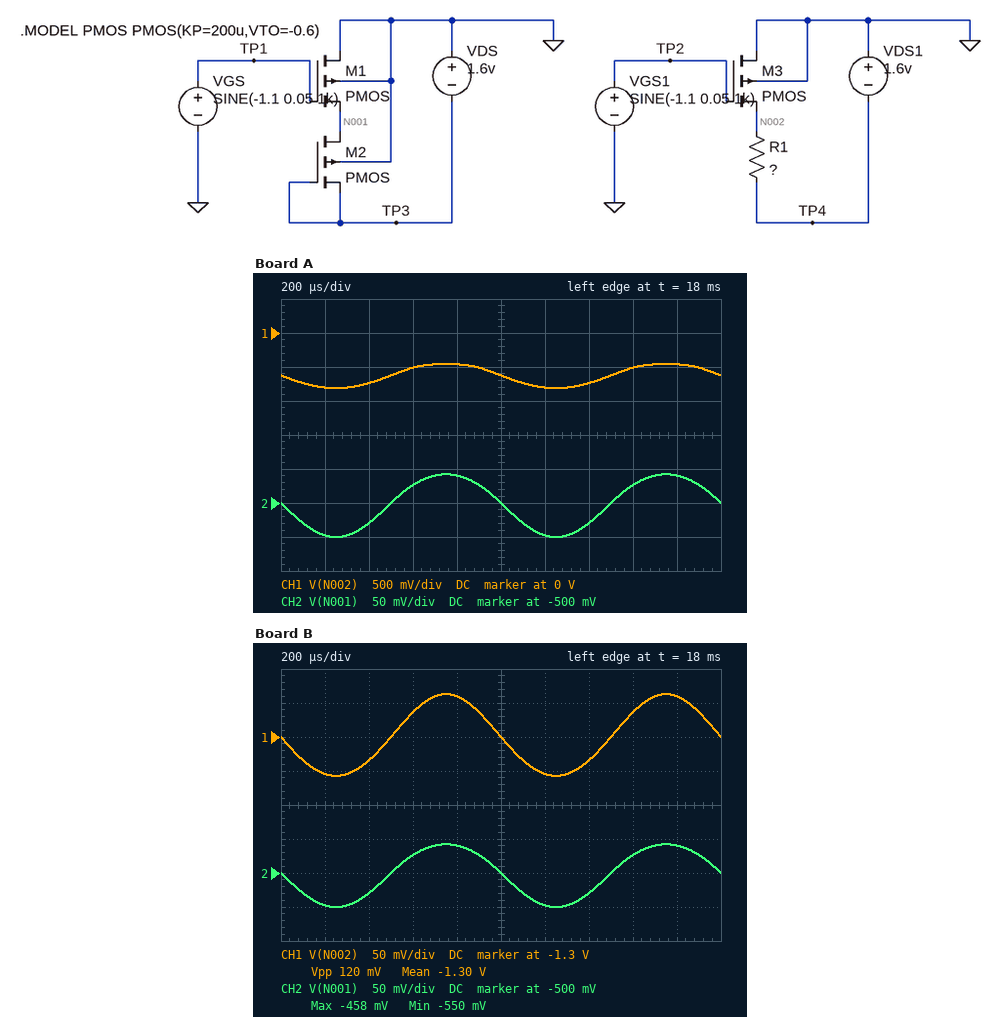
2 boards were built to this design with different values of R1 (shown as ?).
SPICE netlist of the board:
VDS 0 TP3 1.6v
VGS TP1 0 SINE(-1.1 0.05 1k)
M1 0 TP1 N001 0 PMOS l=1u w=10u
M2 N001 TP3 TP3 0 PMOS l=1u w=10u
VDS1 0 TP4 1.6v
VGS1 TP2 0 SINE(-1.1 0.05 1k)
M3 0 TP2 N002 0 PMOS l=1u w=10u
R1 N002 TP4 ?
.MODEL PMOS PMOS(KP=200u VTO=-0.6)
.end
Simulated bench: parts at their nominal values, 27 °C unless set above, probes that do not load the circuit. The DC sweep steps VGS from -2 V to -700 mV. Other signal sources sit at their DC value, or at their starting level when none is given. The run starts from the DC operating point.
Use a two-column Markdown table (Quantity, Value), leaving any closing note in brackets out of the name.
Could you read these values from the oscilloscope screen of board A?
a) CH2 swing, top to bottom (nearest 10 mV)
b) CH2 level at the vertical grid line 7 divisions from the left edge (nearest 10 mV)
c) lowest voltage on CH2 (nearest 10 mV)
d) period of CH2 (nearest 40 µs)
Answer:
| Quantity | Value |
|---|---|
| CH2 swing, top to bottom | 90 mV |
| CH2 level at the vertical grid line 7 divisions from the left edge | -530 mV |
| lowest voltage on CH2 | -550 mV |
| period of CH2 | 1.00 ms |
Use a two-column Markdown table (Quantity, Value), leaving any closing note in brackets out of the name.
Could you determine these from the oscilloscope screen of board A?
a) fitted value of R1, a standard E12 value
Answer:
| Quantity | Value |
|---|---|
| fitted value of R1, a standard E12 value | 3.9 kΩ |
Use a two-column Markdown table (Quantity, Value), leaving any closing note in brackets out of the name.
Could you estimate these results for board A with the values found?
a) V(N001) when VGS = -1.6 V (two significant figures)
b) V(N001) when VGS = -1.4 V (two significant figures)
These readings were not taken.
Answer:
| Quantity | Value |
|---|---|
| V(N001) when VGS = -1.6 V | -290 mV |
| V(N001) when VGS = -1.4 V | -340 mV |
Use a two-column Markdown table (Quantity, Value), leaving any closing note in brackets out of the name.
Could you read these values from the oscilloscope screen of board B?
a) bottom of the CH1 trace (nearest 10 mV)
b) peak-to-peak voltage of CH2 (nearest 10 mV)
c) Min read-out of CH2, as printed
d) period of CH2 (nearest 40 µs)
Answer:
| Quantity | Value |
|---|---|
| bottom of the CH1 trace | -1.36 V |
| peak-to-peak voltage of CH2 | 90 mV |
| Min read-out of CH2, as printed | -550 mV |
| period of CH2 | 1.00 ms |
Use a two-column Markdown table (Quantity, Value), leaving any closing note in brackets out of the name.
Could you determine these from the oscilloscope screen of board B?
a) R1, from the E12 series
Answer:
| Quantity | Value |
|---|---|
| R1, from the E12 series | 1.2 kΩ |
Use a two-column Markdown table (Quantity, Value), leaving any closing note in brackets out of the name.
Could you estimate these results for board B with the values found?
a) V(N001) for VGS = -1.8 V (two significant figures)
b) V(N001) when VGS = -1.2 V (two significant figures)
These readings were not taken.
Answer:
| Quantity | Value |
|---|---|
| V(N001) for VGS = -1.8 V | -260 mV |
| V(N001) when VGS = -1.2 V | -430 mV |
